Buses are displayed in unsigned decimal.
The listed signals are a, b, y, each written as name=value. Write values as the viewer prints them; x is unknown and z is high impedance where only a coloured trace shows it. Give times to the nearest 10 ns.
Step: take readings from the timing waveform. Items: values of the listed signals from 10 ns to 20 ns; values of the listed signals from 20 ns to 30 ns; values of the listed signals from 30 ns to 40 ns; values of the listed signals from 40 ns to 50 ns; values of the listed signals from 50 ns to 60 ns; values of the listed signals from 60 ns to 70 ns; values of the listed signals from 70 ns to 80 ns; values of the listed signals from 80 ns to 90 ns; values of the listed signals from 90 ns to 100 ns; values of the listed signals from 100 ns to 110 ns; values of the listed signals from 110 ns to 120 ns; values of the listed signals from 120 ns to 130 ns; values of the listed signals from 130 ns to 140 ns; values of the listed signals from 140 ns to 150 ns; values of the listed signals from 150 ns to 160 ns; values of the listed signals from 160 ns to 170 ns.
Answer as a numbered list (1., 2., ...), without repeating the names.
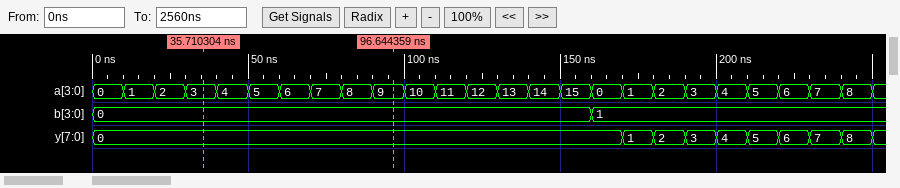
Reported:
1. a=1, b=0, y=0
2. a=2, b=0, y=0
3. a=3, b=0, y=0
4. a=4, b=0, y=0
5. a=5, b=0, y=0
6. a=6, b=0, y=0
7. a=7, b=0, y=0
8. a=8, b=0, y=0
9. a=9, b=0, y=0
10. a=10, b=0, y=0
11. a=11, b=0, y=0
12. a=12, b=0, y=0
13. a=13, b=0, y=0
14. a=14, b=0, y=0
15. a=15, b=0, y=0
16. a=0, b=1, y=0
